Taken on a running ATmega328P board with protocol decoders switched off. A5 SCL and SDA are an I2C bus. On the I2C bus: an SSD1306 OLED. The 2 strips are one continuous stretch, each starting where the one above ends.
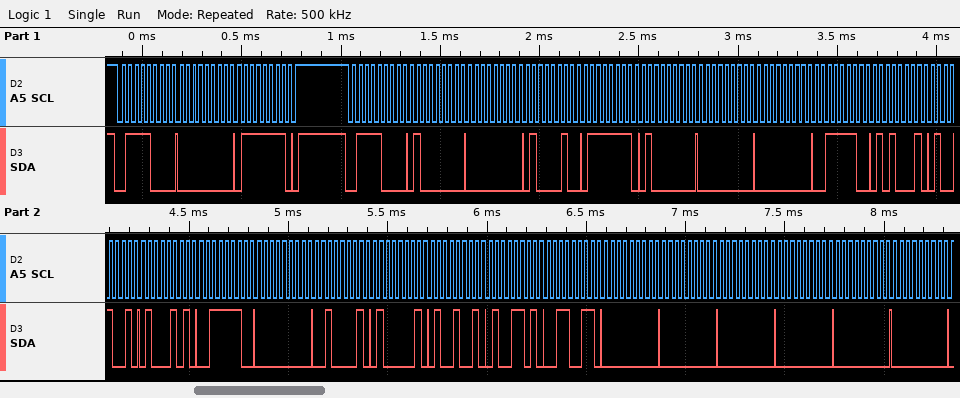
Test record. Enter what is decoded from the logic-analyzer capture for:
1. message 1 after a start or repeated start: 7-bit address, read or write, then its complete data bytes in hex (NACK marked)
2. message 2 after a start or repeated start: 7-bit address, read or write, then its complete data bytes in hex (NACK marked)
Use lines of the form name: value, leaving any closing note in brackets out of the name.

message 1 after a start or repeated start: 7-bit address, read or write, then its complete data bytes in hex: 0x3C write: 00 7F
message 2 after a start or repeated start: 7-bit address, read or write, then its complete data bytes in hex: 0x3C write: 40 00 42 7F 40 00 00 3E 51 49 45 3E 00 21 41 49 4D 33 00 00 00 00 00 00
